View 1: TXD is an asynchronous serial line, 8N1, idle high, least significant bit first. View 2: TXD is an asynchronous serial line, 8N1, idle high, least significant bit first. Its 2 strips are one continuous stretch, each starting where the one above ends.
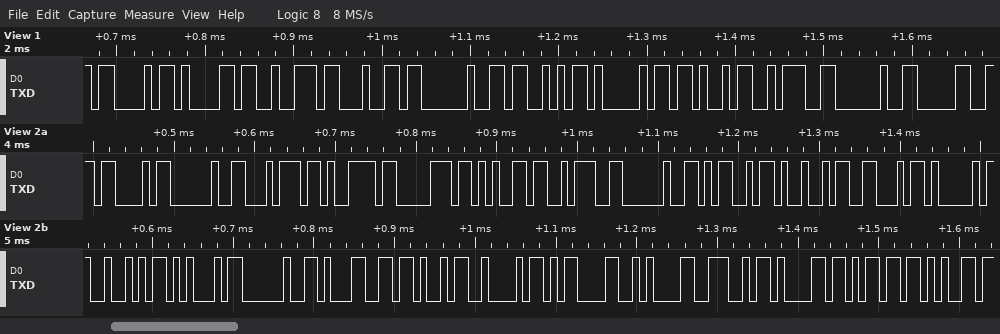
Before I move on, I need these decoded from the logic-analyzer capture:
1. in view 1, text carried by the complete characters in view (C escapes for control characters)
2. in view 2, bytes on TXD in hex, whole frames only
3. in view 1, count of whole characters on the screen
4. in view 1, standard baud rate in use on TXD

"Card SAK: 0"
43 20 74 79 70 65 3A 20 4D 49 46 41 52 45 20 31 4B 42 0D 0A 4E 61 6D 65
11
115200 baud
